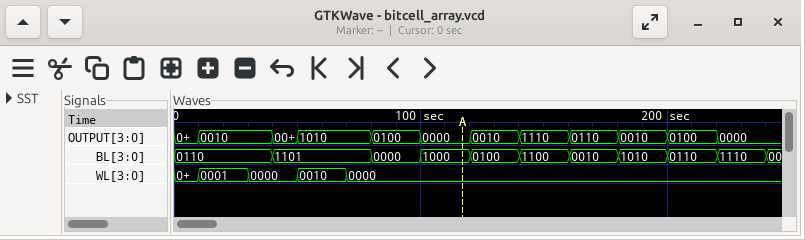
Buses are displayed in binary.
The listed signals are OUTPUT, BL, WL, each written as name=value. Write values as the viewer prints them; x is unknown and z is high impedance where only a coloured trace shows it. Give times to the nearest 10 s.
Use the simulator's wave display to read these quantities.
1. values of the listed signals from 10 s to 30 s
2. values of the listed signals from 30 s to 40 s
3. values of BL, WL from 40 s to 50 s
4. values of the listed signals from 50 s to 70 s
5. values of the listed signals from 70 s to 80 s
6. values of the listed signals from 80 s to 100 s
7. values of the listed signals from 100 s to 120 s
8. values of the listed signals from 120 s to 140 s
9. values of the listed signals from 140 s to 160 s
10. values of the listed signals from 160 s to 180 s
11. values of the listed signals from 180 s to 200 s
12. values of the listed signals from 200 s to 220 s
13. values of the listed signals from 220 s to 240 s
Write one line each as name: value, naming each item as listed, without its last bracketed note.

values of the listed signals from 10 s to 30 s: OUTPUT=0010, BL=0110, WL=0001
values of the listed signals from 30 s to 40 s: OUTPUT=0010, BL=0110, WL=0000
values of BL, WL from 40 s to 50 s: BL=1101, WL=0000
values of the listed signals from 50 s to 70 s: OUTPUT=1010, BL=1101, WL=0010
values of the listed signals from 70 s to 80 s: OUTPUT=1010, BL=1101, WL=0000
values of the listed signals from 80 s to 100 s: OUTPUT=0100, BL=0000, WL=0000
values of the listed signals from 100 s to 120 s: OUTPUT=0000, BL=1000, WL=0000
values of the listed signals from 120 s to 140 s: OUTPUT=0010, BL=0100, WL=0000
values of the listed signals from 140 s to 160 s: OUTPUT=1110, BL=1100, WL=0000
values of the listed signals from 160 s to 180 s: OUTPUT=0110, BL=0010, WL=0000
values of the listed signals from 180 s to 200 s: OUTPUT=0010, BL=1010, WL=0000
values of the listed signals from 200 s to 220 s: OUTPUT=0100, BL=0110, WL=0000
values of the listed signals from 220 s to 240 s: OUTPUT=0000, BL=1110, WL=0000
